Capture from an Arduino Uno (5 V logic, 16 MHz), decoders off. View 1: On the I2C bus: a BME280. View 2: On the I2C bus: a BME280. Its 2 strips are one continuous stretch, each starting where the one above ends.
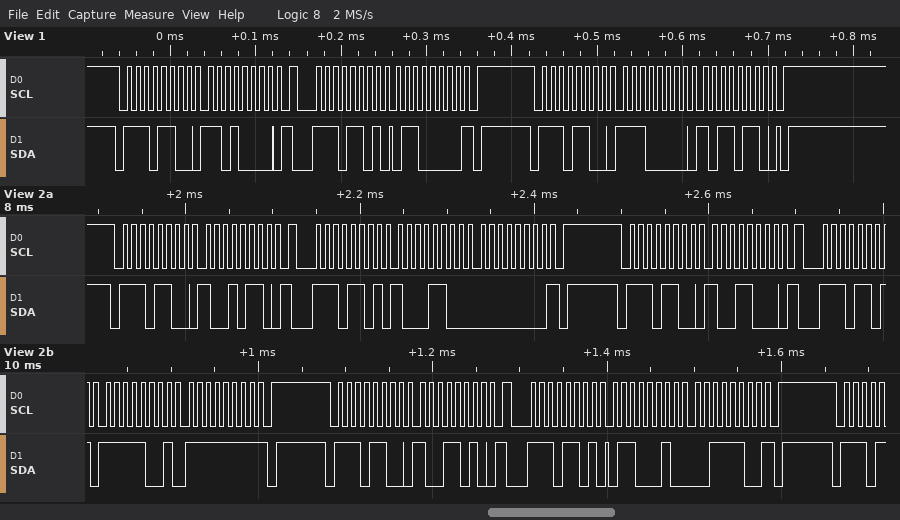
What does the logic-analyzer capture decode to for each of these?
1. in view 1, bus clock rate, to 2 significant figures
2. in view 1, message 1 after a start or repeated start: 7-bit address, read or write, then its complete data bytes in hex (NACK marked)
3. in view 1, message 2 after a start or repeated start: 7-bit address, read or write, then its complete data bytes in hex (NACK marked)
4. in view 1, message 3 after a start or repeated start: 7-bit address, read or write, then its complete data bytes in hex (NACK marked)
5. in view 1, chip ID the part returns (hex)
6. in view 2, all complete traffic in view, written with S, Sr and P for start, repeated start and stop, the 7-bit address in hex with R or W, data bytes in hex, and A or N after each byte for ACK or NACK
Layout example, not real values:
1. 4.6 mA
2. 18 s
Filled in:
1. 100 kHz
2. 0x76 write: D0
3. 0x76 read: 60 NACK
4. 0x76 write: E0 B6
5. 0x60
6. S 76W A 96 A Sr 76R A 8C A 00 N P S 76W A 98 A Sr 76R A F9 A FF N P S 76W A 9A A Sr 76R A 62 A 3C N P
